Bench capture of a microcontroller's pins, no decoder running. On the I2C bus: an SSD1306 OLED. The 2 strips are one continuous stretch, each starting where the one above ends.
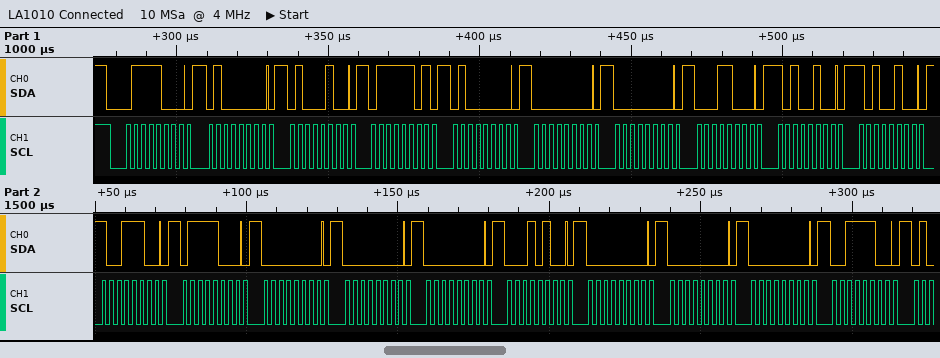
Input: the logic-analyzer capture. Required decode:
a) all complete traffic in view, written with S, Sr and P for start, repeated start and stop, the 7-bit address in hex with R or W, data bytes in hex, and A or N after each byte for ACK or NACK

S 3CW A 40 A 44 A 7D A 40 A 00 A 00 A 18 A A4 A A4 A 9C A 78 A 00 A 00 A 00 A 14 A 00 A 00 A 00 A 3C A
